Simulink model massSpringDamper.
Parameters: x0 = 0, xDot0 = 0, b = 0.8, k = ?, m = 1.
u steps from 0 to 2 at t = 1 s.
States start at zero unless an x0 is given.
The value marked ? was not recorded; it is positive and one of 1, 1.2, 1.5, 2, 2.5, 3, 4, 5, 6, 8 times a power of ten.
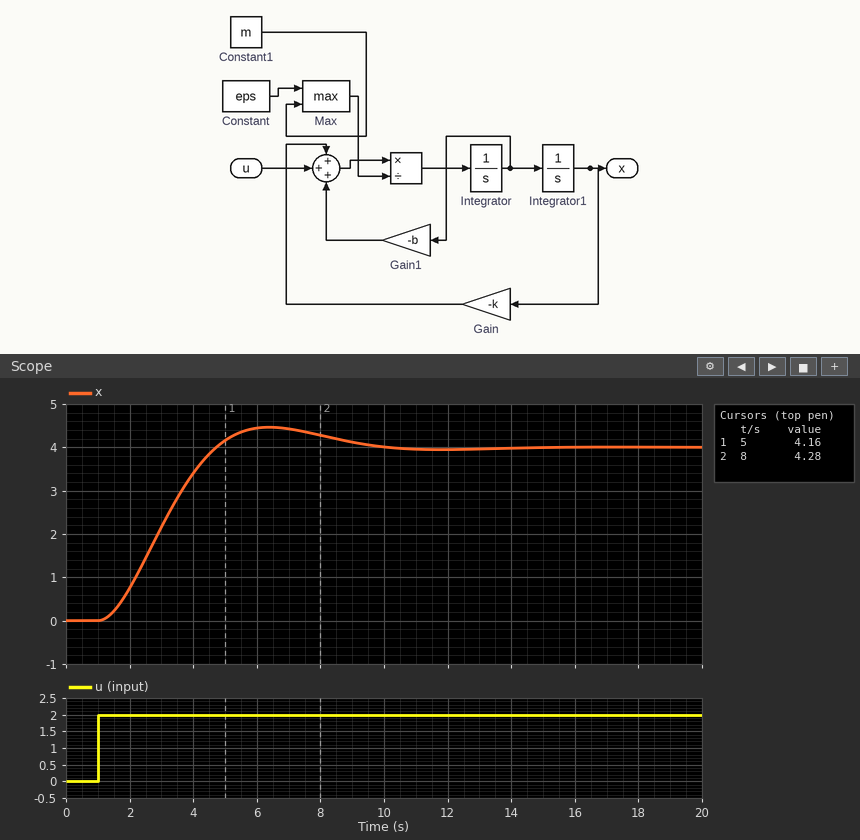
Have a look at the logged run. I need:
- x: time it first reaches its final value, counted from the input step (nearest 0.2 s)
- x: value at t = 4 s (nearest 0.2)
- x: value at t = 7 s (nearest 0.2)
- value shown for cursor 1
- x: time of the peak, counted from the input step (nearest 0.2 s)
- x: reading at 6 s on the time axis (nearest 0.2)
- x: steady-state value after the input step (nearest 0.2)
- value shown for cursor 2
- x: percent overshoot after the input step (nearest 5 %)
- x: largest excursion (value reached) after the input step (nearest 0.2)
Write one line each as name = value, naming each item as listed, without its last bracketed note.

x: time it first reaches its final value, counted from the input step = 3.8 s
x: value at t = 4 s = 3.4
x: value at t = 7 s = 4.4
value shown for cursor 1 = 4.16
x: time of the peak, counted from the input step = 5.4 s
x: reading at 6 s on the time axis = 4.4
x: steady-state value after the input step = 4.0
value shown for cursor 2 = 4.28
x: percent overshoot after the input step = 10 %
x: largest excursion (value reached) after the input step = 4.4
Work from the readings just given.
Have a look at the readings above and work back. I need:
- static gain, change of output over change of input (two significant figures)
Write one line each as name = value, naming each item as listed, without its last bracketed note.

static gain, change of output over change of input = 2.0
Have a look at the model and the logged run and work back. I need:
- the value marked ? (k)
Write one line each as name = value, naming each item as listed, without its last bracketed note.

the value marked ? = 0.5
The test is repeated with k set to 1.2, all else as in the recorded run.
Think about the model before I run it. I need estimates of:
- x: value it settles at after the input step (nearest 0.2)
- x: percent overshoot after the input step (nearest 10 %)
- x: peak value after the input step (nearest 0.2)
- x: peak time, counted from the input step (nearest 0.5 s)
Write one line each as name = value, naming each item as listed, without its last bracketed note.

x: value it settles at after the input step = 1.6
x: percent overshoot after the input step = 30 %
x: peak value after the input step = 2.2
x: peak time, counted from the input step = 3.0 s
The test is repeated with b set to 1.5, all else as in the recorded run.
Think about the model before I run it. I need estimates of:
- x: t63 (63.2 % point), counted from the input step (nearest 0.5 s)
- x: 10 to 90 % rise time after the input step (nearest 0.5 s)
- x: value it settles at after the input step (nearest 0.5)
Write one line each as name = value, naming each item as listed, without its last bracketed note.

x: t63 (63.2 % point), counted from the input step = 3.0 s
x: 10 to 90 % rise time after the input step = 5.0 s
x: value it settles at after the input step = 4.0
